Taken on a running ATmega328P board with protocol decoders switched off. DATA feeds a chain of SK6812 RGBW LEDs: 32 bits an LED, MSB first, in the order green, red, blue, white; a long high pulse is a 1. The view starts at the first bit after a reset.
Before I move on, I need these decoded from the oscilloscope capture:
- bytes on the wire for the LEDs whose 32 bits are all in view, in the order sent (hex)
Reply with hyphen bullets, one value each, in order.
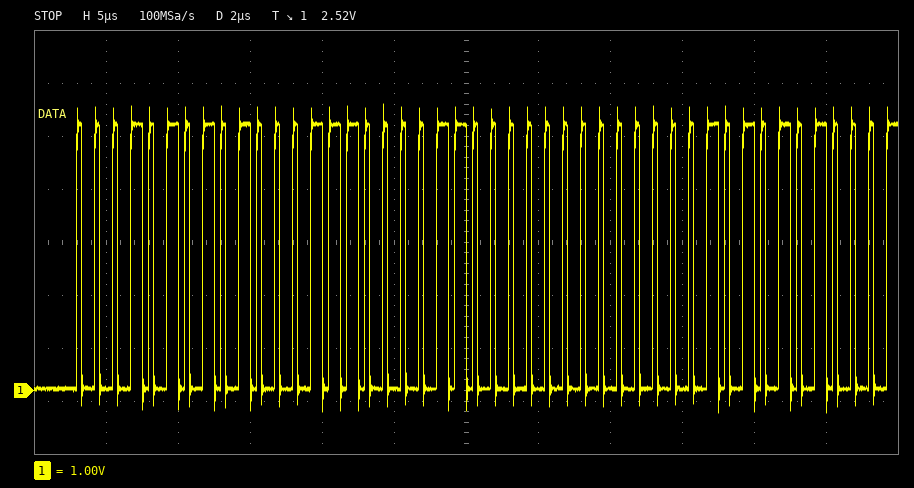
- 15 47 0C 00
